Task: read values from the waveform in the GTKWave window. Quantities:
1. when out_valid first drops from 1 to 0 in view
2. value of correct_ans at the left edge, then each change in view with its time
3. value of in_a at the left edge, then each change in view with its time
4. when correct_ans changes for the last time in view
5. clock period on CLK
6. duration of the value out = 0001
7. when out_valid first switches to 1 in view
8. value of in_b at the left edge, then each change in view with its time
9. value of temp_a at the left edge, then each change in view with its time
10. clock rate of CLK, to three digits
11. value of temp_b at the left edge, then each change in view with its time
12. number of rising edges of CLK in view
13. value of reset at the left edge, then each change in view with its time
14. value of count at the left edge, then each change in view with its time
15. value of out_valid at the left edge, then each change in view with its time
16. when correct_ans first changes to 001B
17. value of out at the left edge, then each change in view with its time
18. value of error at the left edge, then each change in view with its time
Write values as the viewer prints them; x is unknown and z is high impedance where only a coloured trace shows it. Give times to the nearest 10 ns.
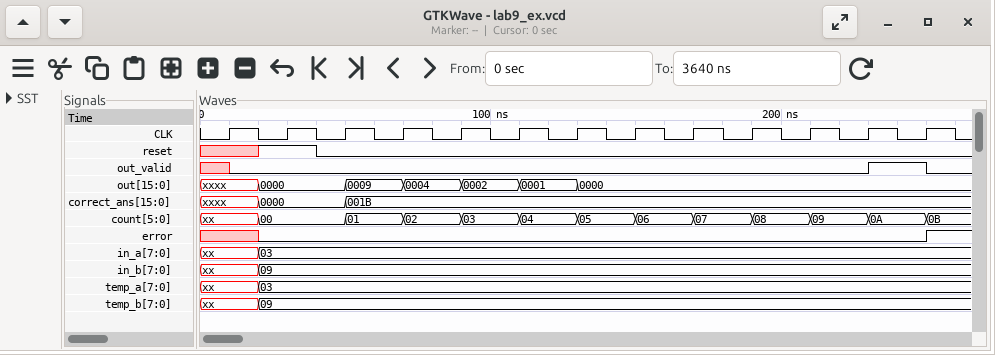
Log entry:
250 ns
xxxx, 0000 at 20 ns, 001B at 50 ns
xx, 03 at 20 ns
50 ns
20 ns
20 ns
230 ns
xx, 09 at 20 ns
xx, 03 at 20 ns
50.0 MHz
xx, 09 at 20 ns
13
x, 1 at 20 ns, 0 at 40 ns
xx, 00 at 20 ns, 01 at 50 ns, 02 at 70 ns, 03 at 90 ns, 04 at 110 ns, 05 at 130 ns, 06 at 150 ns, 07 at 170 ns, 08 at 190 ns, 09 at 210 ns, 0A at 230 ns, 0B at 250 ns
x, 0 at 10 ns, 1 at 230 ns, 0 at 250 ns
50 ns
xxxx, 0000 at 20 ns, 0009 at 50 ns, 0004 at 70 ns, 0002 at 90 ns, 0001 at 110 ns, 0000 at 130 ns
x, 0 at 20 ns, 1 at 250 ns
